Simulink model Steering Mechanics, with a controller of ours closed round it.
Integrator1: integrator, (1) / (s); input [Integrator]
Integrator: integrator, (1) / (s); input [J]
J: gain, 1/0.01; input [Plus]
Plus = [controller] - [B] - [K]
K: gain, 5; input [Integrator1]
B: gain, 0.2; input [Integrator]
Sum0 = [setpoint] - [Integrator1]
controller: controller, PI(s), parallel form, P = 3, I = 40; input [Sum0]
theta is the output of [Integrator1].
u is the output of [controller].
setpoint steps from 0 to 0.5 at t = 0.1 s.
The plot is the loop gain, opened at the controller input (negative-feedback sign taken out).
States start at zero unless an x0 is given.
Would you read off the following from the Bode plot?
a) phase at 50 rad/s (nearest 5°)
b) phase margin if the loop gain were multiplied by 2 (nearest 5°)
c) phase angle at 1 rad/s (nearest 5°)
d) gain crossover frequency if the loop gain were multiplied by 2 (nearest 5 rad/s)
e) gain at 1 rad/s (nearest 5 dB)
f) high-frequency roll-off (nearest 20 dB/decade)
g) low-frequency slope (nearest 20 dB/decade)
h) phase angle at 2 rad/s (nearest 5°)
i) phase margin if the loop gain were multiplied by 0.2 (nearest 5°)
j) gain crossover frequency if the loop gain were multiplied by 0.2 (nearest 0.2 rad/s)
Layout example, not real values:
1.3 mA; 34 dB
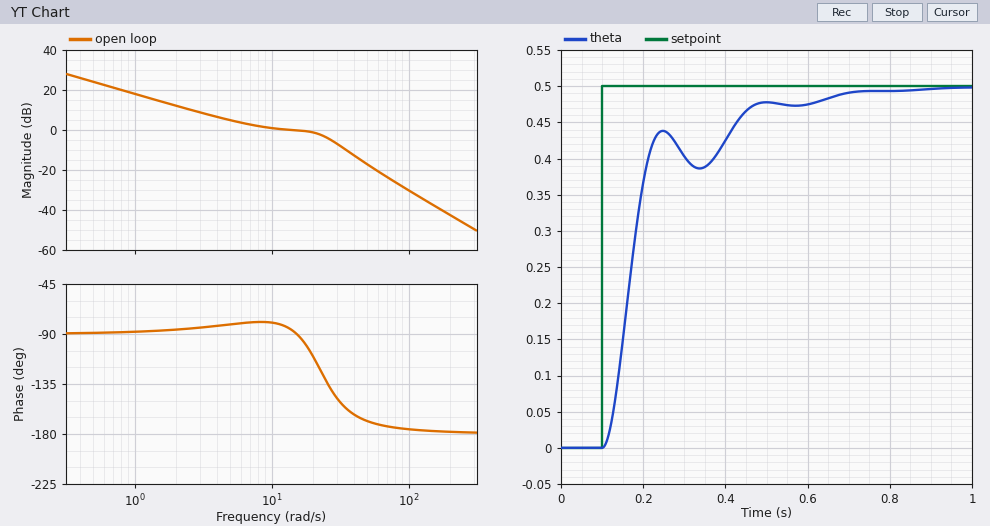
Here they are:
-170°; 35°; -90°; 30 rad/s; 20 dB; -40 dB/decade; -20 dB/decade; -85°; 95°; 1.6 rad/s
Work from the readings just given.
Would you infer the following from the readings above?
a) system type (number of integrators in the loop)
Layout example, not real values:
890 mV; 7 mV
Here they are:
1
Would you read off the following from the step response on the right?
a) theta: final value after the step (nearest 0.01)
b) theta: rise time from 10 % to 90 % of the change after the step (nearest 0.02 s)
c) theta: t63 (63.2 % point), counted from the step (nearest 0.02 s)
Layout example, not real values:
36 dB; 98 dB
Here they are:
0.50; 0.30 s; 0.08 s
